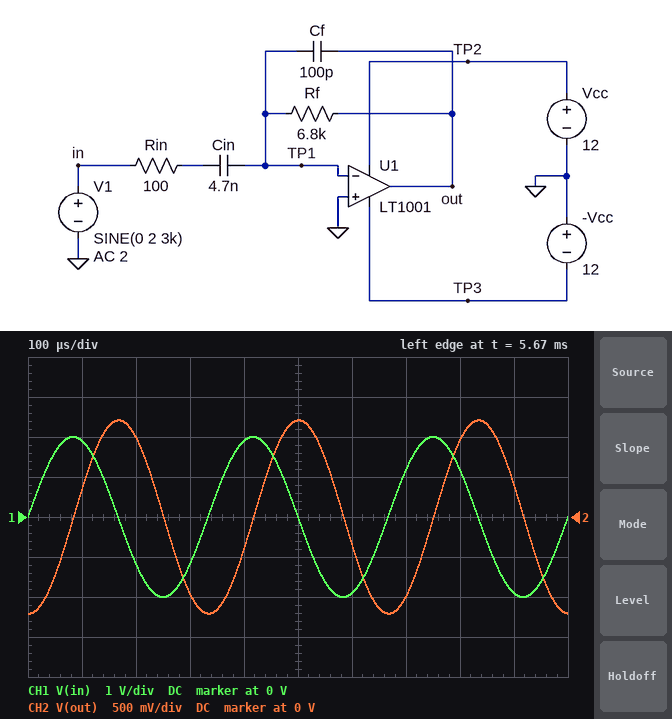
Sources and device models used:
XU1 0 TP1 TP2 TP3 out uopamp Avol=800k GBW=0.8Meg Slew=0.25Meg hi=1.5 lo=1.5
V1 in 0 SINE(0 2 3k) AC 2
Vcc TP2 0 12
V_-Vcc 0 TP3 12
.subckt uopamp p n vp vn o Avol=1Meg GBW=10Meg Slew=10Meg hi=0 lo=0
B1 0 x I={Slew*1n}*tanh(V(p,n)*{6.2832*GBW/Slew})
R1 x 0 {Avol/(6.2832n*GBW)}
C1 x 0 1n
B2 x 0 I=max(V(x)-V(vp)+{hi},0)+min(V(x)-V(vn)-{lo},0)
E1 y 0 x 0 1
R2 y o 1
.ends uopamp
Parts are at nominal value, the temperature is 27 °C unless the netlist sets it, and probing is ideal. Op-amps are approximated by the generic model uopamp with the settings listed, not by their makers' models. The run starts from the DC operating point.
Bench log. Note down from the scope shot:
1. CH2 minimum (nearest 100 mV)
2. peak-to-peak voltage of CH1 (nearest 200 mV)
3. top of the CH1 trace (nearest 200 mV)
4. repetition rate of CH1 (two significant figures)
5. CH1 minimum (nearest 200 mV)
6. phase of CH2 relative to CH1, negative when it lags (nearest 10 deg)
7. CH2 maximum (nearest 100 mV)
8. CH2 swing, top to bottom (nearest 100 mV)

-1.2 V
4.0 V
2.0 V
3.0 kHz
-2.0 V
-90 deg
1.2 V
2.4 V
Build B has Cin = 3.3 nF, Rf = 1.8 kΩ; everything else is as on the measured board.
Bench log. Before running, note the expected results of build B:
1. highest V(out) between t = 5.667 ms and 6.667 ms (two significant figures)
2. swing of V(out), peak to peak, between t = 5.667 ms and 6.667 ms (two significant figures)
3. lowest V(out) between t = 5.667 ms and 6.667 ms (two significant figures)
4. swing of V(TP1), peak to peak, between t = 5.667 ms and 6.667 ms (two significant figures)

220 mV
450 mV
-220 mV
1.7 mV
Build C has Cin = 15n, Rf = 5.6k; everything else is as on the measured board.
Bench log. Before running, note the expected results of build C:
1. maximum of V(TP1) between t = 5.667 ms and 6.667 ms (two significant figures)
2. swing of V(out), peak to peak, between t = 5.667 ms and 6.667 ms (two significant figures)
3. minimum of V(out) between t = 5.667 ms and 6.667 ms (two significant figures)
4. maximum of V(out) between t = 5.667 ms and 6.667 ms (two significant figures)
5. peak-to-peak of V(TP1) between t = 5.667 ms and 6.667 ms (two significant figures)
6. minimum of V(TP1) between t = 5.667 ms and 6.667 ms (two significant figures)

12 mV
6.4 V
-3.2 V
3.2 V
24 mV
-12 mV
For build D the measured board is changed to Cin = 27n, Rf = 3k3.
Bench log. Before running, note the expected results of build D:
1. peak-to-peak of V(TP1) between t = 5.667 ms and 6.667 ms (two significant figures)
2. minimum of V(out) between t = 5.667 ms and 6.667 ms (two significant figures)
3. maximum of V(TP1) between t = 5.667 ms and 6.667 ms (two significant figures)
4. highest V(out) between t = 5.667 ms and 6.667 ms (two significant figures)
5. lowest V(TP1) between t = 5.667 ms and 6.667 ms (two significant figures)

26 mV
-3.4 V
13 mV
3.4 V
-13 mV
